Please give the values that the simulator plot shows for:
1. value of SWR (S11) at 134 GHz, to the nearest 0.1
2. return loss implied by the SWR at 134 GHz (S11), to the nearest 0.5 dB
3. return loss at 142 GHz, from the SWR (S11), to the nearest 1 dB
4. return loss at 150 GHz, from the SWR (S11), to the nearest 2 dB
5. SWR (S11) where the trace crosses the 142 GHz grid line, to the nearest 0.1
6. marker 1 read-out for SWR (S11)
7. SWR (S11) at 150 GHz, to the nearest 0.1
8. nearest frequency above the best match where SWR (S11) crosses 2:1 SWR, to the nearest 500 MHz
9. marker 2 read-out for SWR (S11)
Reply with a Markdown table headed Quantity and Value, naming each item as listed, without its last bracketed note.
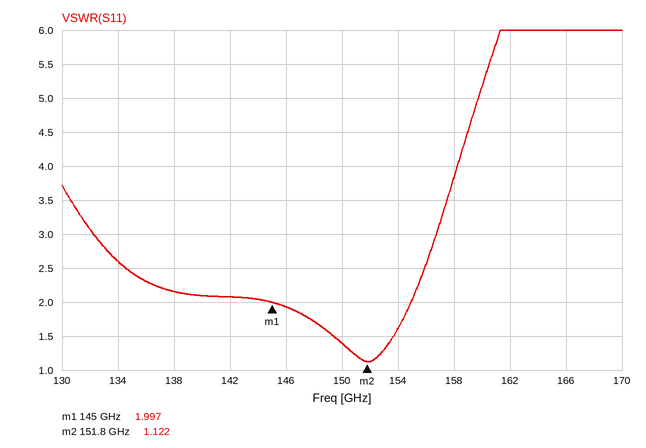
| Quantity | Value |
|---|---|
| value of SWR (S11) at 134 GHz, to the nearest 0.1 | 2.6 |
| return loss implied by the SWR at 134 GHz (S11), to the nearest 0.5 dB | 7.0 dB |
| return loss at 142 GHz, from the SWR (S11), to the nearest 1 dB | 9 dB |
| return loss at 150 GHz, from the SWR (S11), to the nearest 2 dB | 16 dB |
| SWR (S11) where the trace crosses the 142 GHz grid line, to the nearest 0.1 | 2.1 |
| marker 1 read-out for SWR | 1.997 |
| SWR (S11) at 150 GHz, to the nearest 0.1 | 1.4 |
| nearest frequency above the best match where SWR (S11) crosses 2:1 SWR, to the nearest 500 MHz | 155.0 GHz |
| marker 2 read-out for SWR | 1.122 |
